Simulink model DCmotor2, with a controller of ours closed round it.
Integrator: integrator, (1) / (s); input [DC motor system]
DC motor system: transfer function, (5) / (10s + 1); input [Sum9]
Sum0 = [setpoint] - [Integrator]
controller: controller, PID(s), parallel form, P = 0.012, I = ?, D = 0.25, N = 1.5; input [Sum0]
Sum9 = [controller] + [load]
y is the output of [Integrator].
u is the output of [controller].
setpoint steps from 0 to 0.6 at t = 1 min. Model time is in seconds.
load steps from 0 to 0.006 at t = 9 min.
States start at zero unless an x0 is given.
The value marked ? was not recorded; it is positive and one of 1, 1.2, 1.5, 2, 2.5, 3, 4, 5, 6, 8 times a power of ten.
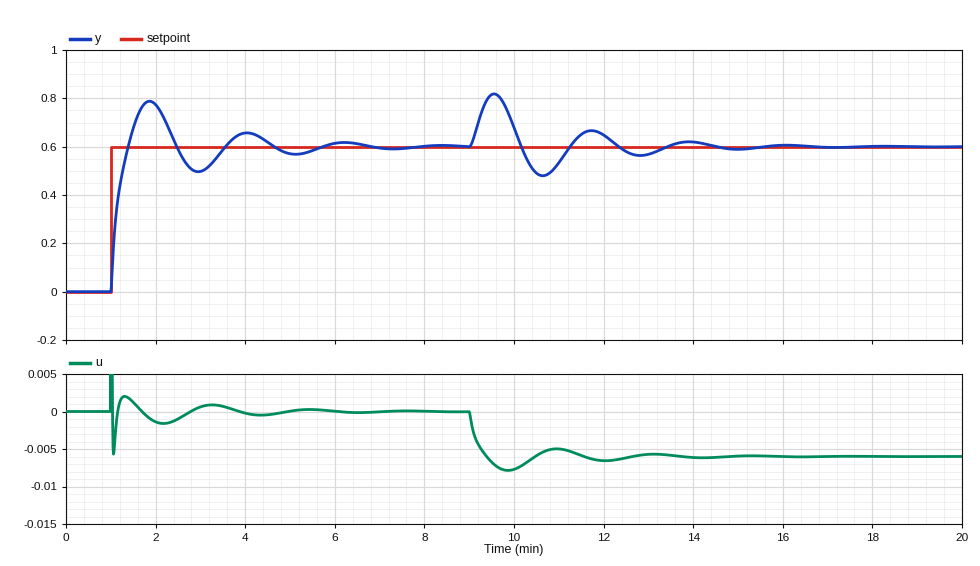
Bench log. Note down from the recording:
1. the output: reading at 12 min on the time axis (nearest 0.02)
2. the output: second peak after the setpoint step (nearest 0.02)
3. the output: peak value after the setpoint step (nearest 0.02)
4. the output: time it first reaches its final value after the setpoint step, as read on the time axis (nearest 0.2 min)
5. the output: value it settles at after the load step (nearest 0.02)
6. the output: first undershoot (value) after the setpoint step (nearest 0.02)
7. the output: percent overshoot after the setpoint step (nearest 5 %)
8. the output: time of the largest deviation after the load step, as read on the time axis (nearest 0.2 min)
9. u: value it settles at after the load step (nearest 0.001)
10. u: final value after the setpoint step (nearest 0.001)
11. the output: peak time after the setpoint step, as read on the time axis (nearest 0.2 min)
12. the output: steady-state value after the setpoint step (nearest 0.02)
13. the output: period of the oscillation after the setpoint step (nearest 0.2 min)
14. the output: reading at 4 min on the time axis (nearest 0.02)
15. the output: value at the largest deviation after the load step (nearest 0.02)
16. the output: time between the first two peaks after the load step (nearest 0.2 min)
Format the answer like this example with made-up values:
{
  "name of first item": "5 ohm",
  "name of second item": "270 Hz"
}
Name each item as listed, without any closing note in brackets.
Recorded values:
{
  "the output: reading at 12 min on the time axis": "0.64",
  "the output: second peak after the setpoint step": "0.66",
  "the output: peak value after the setpoint step": "0.78",
  "the output: time it first reaches its final value after the setpoint step, as read on the time axis": "1.4 min",
  "the output: value it settles at after the load step": "0.60",
  "the output: first undershoot (value) after the setpoint step": "0.50",
  "the output: percent overshoot after the setpoint step": "30 %",
  "the output: time of the largest deviation after the load step, as read on the time axis": "9.6 min",
  "u: value it settles at after the load step": "-0.006",
  "u: final value after the setpoint step": "0.000",
  "the output: peak time after the setpoint step, as read on the time axis": "1.8 min",
  "the output: steady-state value after the setpoint step": "0.60",
  "the output: period of the oscillation after the setpoint step": "2.2 min",
  "the output: reading at 4 min on the time axis": "0.66",
  "the output: value at the largest deviation after the load step": "0.82",
  "the output: time between the first two peaks after the load step": "2.2 min"
}
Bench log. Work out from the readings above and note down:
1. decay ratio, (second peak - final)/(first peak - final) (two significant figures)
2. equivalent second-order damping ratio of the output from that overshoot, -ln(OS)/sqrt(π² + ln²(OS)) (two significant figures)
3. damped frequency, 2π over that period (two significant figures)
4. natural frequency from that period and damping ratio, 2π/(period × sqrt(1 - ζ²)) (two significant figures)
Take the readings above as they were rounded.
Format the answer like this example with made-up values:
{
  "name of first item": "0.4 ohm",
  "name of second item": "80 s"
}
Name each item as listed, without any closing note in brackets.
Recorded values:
{
  "decay ratio, (second peak - final)/(first peak - final)": "0.33",
  "equivalent second-order damping ratio of the output from that overshoot, -ln(OS)/sqrt(π² + ln²(OS))": "0.36",
  "damped frequency, 2π over that period": "2.9 rad/min",
  "natural frequency from that period and damping ratio, 2π/(period × sqrt(1 - ζ²))": "3.1 rad/min"
}
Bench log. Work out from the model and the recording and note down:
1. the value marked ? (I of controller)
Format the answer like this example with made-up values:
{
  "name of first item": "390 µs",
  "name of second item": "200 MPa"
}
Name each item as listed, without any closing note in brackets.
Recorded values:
{
  "the value marked ?": "0.001"
}
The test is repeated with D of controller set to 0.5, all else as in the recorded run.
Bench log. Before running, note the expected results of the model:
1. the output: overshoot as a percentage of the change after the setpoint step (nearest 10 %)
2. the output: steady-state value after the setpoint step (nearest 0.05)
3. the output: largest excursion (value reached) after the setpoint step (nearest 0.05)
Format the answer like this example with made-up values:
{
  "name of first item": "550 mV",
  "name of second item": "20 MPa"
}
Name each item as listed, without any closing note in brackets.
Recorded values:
{
  "the output: overshoot as a percentage of the change after the setpoint step": "20 %",
  "the output: steady-state value after the setpoint step": "0.60",
  "the output: largest excursion (value reached) after the setpoint step": "0.70"
}
